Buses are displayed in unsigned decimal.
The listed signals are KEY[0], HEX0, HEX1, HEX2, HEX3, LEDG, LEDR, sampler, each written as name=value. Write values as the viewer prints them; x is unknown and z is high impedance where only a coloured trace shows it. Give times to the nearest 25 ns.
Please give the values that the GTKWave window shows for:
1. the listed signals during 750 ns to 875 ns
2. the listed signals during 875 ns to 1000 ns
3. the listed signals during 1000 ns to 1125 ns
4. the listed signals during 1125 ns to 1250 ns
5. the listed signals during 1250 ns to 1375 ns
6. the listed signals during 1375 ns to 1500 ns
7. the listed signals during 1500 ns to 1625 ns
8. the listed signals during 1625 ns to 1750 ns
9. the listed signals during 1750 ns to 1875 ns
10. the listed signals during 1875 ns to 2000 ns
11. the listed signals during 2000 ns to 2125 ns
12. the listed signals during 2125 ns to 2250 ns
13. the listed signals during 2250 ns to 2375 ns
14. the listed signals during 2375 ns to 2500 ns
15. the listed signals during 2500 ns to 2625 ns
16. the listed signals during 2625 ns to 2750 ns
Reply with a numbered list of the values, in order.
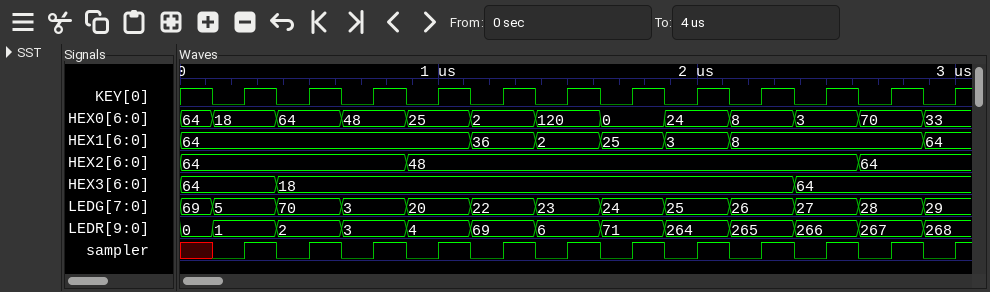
1. KEY[0]=1, HEX0=48, HEX1=64, HEX2=64, HEX3=18, LEDG=3, LEDR=3, sampler=1
2. KEY[0]=0, HEX0=25, HEX1=64, HEX2=48, HEX3=18, LEDG=20, LEDR=4, sampler=0
3. KEY[0]=1, HEX0=25, HEX1=64, HEX2=48, HEX3=18, LEDG=20, LEDR=4, sampler=1
4. KEY[0]=0, HEX0=2, HEX1=36, HEX2=48, HEX3=18, LEDG=22, LEDR=69, sampler=0
5. KEY[0]=1, HEX0=2, HEX1=36, HEX2=48, HEX3=18, LEDG=22, LEDR=69, sampler=1
6. KEY[0]=0, HEX0=120, HEX1=2, HEX2=48, HEX3=18, LEDG=23, LEDR=6, sampler=0
7. KEY[0]=1, HEX0=120, HEX1=2, HEX2=48, HEX3=18, LEDG=23, LEDR=6, sampler=1
8. KEY[0]=0, HEX0=0, HEX1=25, HEX2=48, HEX3=18, LEDG=24, LEDR=71, sampler=0
9. KEY[0]=1, HEX0=0, HEX1=25, HEX2=48, HEX3=18, LEDG=24, LEDR=71, sampler=1
10. KEY[0]=0, HEX0=24, HEX1=3, HEX2=48, HEX3=18, LEDG=25, LEDR=264, sampler=0
11. KEY[0]=1, HEX0=24, HEX1=3, HEX2=48, HEX3=18, LEDG=25, LEDR=264, sampler=1
12. KEY[0]=0, HEX0=8, HEX1=8, HEX2=48, HEX3=18, LEDG=26, LEDR=265, sampler=0
13. KEY[0]=1, HEX0=8, HEX1=8, HEX2=48, HEX3=18, LEDG=26, LEDR=265, sampler=1
14. KEY[0]=0, HEX0=3, HEX1=8, HEX2=48, HEX3=64, LEDG=27, LEDR=266, sampler=0
15. KEY[0]=1, HEX0=3, HEX1=8, HEX2=48, HEX3=64, LEDG=27, LEDR=266, sampler=1
16. KEY[0]=0, HEX0=70, HEX1=8, HEX2=64, HEX3=64, LEDG=28, LEDR=267, sampler=0
